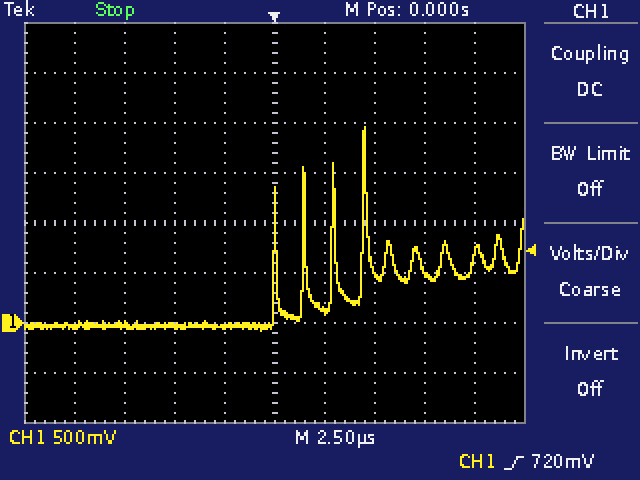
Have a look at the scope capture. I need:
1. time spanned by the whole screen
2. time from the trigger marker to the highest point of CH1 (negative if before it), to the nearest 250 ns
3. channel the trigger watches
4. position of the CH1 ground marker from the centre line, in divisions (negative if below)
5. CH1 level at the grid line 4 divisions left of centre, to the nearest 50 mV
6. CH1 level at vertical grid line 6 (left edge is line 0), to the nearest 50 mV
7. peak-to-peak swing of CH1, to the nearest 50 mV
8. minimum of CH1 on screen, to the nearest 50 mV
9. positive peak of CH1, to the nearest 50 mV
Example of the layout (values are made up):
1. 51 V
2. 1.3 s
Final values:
1. 25 µs
2. +4.50 µs
3. CH1
4. -2.0 div
5. -50 mV
6. 100 mV
7. 2.05 V
8. -100 mV
9. 1.95 V
